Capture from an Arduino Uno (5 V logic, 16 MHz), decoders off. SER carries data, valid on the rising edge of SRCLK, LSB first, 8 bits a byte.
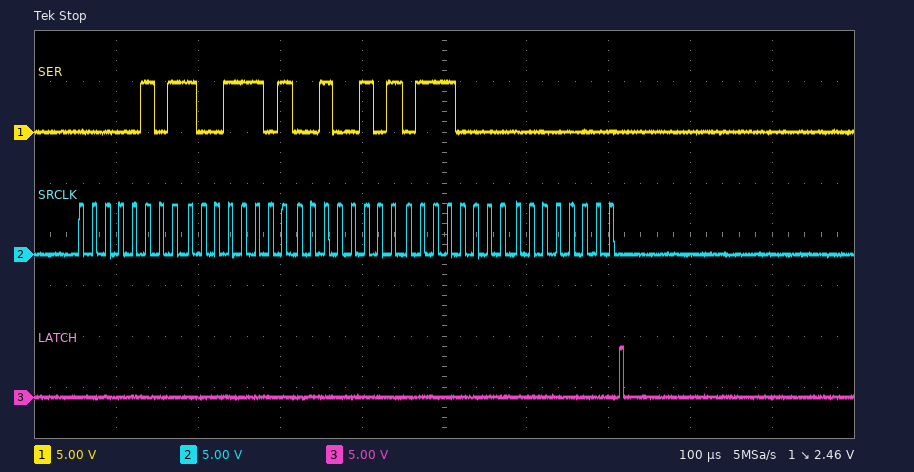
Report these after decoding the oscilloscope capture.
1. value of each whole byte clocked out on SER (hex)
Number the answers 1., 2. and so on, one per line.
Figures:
1. 0xA0 0xB9 0xA4 0x0E 0x00
